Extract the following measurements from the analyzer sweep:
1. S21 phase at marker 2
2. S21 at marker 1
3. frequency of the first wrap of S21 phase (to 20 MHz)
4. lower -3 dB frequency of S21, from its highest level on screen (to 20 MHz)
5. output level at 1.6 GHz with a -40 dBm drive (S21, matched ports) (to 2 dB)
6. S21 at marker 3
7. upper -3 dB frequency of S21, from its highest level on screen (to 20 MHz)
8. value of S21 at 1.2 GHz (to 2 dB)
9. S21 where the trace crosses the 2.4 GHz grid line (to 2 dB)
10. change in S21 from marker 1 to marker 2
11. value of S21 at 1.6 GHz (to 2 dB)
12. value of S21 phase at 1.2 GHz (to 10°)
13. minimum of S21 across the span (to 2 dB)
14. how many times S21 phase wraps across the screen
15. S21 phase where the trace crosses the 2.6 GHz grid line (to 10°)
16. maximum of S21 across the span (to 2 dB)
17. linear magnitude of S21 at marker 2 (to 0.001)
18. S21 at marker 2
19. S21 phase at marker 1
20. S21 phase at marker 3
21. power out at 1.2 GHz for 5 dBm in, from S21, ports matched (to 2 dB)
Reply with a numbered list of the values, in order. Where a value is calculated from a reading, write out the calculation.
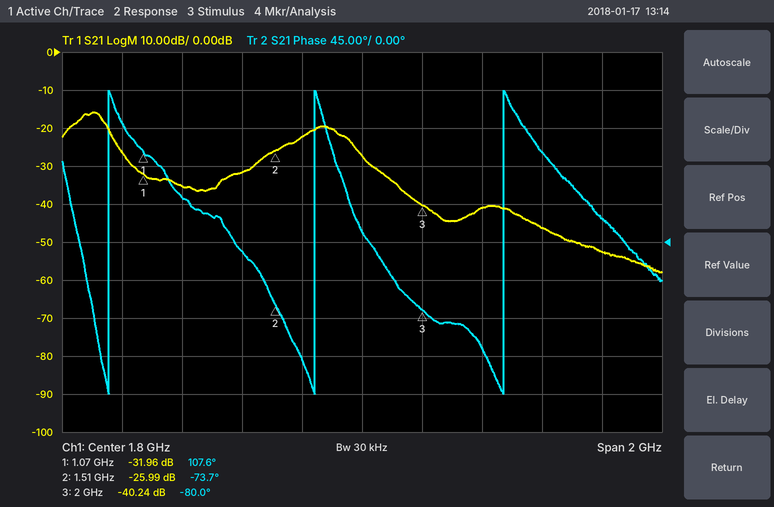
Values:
1. -73.7°
2. -31.96 dB
3. 960 MHz
4. 840 MHz
5. -40 dBm + (-22 dB) = -62 dBm
6. -40.24 dB
7. 940 MHz
8. -36 dB
9. -46 dB
10. -25.99 − (-31.96) = 5.97 dB
11. -22 dB
12. 50°
13. -58 dB
14. 3
15. 30°
16. -16 dB
17. 10^(-25.99/20) ≈ 0.050
18. -25.99 dB
19. 107.6°
20. -80.0°
21. 5 dBm + (-36 dB) = -30 dBm
